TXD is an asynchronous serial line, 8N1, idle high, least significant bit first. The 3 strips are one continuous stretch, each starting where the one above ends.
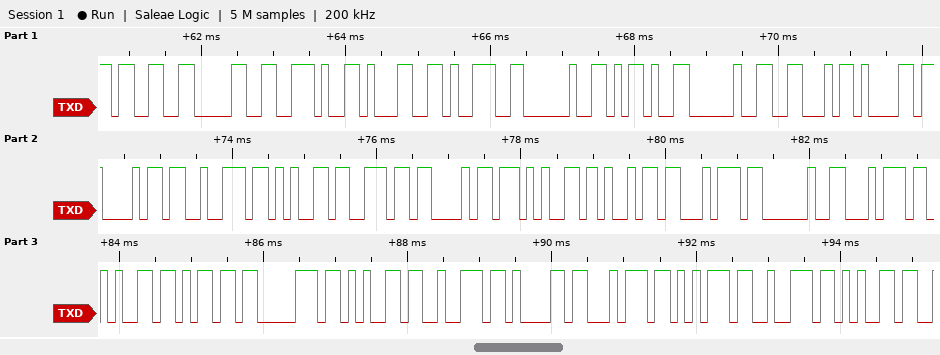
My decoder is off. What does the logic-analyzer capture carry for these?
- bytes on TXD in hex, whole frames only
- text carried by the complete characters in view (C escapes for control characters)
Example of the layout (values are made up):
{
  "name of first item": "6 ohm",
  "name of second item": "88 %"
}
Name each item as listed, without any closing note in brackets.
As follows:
{
  "bytes on TXD in hex, whole frames only": "33 30 2E 31 39 20 2D 20 46 61 68 72 65 6E 68 65 69 74 20 74 65 6D 70 65 72 61 74 75 72 65",
  "text carried by the complete characters in view": "\"30.19 - Fahrenheit temperature\""
}
